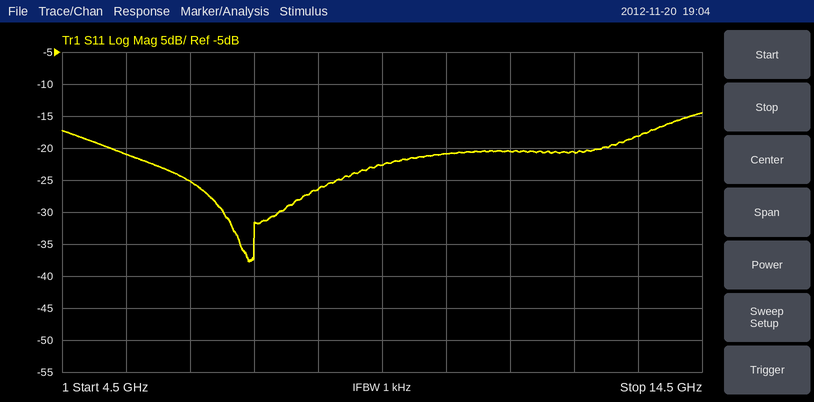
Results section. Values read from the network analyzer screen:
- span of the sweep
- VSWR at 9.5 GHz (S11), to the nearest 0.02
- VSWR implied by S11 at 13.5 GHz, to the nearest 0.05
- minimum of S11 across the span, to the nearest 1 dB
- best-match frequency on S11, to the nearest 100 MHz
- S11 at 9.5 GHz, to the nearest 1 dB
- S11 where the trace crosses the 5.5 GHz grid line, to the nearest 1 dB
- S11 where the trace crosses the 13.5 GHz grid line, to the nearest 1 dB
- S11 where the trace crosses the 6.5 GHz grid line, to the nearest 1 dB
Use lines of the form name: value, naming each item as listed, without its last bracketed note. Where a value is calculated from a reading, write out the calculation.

span of the sweep: 10 GHz
VSWR at 9.5 GHz (S11), to the nearest 0.02: |Γ| = 10^(-23/20) = 0.0708; VSWR = (1 + 0.0708)/(1 − 0.0708) ≈ 1.15, so 1.16 to the nearest 0.02
VSWR implied by S11 at 13.5 GHz, to the nearest 0.05: |Γ| = 10^(-18/20) = 0.1259; VSWR = (1 + 0.1259)/(1 − 0.1259) ≈ 1.29, so 1.30 to the nearest 0.05
minimum of S11 across the span, to the nearest 1 dB: -38 dB
best-match frequency on S11, to the nearest 100 MHz: 7.4 GHz
S11 at 9.5 GHz, to the nearest 1 dB: -23 dB
S11 where the trace crosses the 5.5 GHz grid line, to the nearest 1 dB: -21 dB
S11 where the trace crosses the 13.5 GHz grid line, to the nearest 1 dB: -18 dB
S11 where the trace crosses the 6.5 GHz grid line, to the nearest 1 dB: -25 dB
